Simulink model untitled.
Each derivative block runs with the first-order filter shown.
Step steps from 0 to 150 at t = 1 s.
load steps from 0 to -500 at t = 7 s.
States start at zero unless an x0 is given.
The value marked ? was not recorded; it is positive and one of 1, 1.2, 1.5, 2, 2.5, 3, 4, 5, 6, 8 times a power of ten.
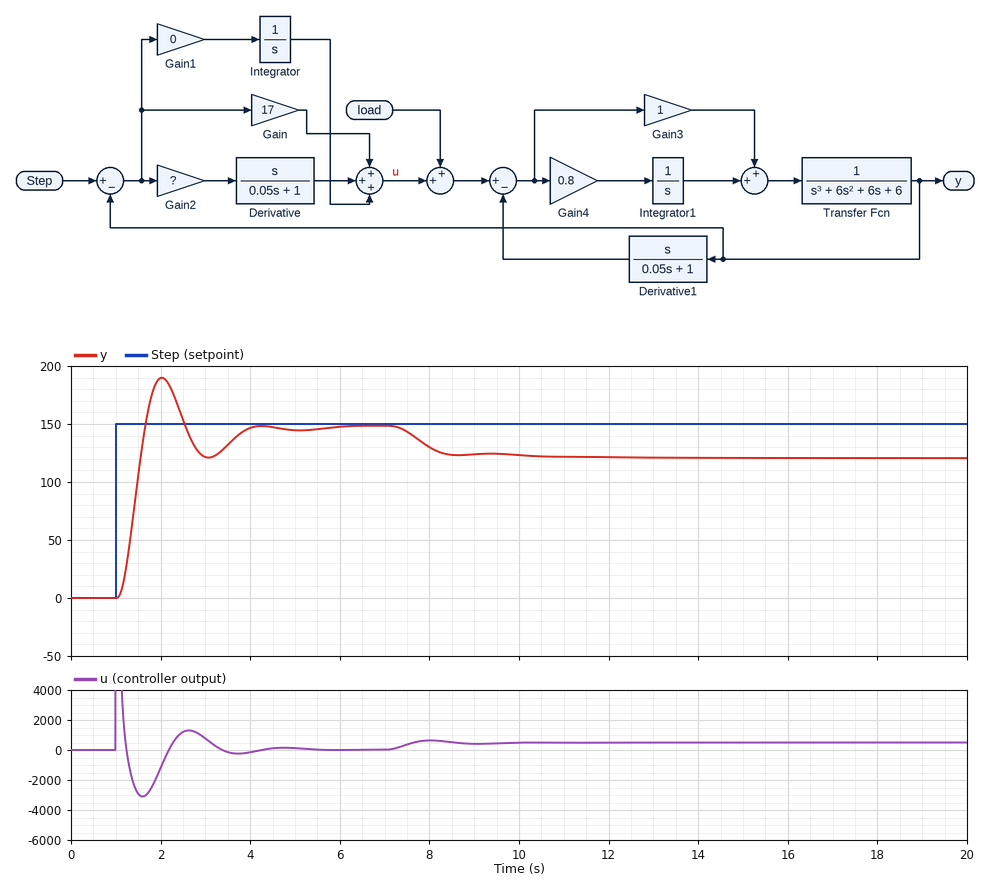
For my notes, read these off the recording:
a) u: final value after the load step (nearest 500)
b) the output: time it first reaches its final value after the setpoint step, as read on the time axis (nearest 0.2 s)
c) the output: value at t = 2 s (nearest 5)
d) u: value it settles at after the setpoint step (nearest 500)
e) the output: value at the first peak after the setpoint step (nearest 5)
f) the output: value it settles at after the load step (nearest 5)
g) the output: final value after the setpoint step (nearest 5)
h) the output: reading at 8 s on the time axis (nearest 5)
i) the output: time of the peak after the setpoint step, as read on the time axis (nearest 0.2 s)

500
1.6 s
190
0
190
120
150
130
2.0 s
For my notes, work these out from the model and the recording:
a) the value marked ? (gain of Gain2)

12
